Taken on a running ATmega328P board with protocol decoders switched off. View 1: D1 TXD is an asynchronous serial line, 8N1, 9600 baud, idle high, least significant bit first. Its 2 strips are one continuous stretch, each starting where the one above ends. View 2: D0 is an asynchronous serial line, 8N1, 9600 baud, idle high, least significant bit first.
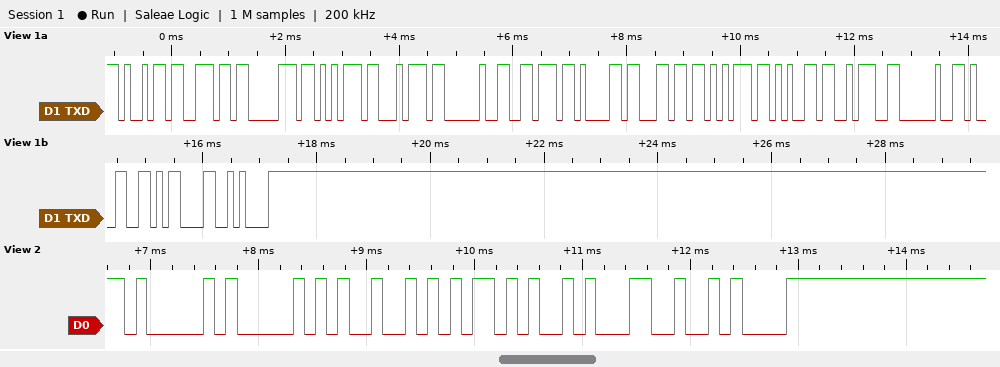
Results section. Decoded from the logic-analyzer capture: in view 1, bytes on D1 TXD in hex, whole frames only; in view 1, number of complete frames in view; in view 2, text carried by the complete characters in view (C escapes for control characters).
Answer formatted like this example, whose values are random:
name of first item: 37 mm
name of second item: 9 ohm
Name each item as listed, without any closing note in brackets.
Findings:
in view 1, bytes on D1 TXD in hex, whole frames only: 69 6E 70 75 74 20 76 61 6C 75 65 3A 20 31 0D 0A
in view 1, number of complete frames in view: 16
in view 2, text carried by the complete characters in view: "APR+1\n"
